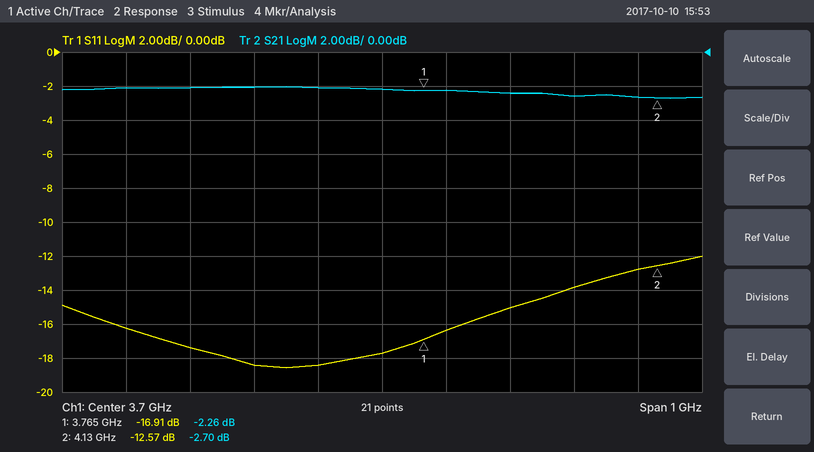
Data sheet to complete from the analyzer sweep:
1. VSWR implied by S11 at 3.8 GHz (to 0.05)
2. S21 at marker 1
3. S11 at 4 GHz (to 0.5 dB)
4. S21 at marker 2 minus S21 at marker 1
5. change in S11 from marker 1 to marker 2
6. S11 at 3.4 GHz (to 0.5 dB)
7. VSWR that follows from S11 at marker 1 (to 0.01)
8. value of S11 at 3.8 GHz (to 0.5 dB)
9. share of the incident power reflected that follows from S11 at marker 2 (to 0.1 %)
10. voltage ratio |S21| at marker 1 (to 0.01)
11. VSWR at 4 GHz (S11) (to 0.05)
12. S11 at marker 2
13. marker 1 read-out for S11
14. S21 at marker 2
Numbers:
1.35
-2.26 dB
-14.0 dB
-0.44 dB
4.34 dB
-17.5 dB
1.33
-16.5 dB
5.5 %
0.77
1.50
-12.57 dB
-16.91 dB
-2.70 dB
